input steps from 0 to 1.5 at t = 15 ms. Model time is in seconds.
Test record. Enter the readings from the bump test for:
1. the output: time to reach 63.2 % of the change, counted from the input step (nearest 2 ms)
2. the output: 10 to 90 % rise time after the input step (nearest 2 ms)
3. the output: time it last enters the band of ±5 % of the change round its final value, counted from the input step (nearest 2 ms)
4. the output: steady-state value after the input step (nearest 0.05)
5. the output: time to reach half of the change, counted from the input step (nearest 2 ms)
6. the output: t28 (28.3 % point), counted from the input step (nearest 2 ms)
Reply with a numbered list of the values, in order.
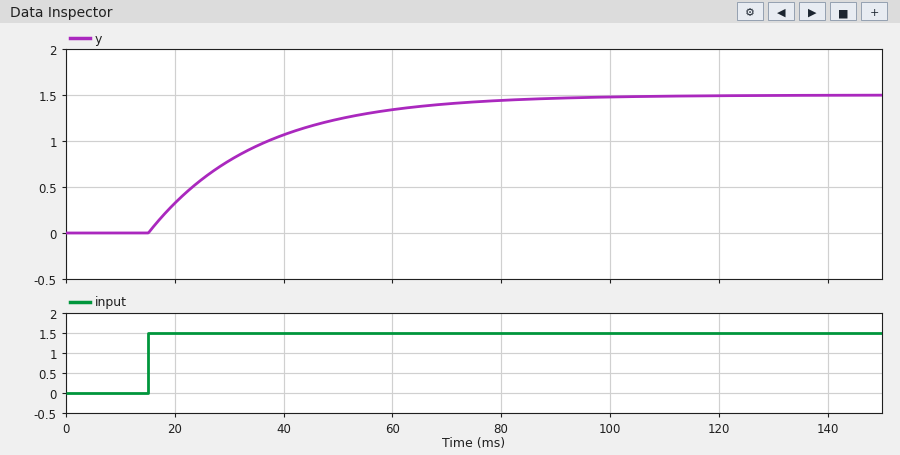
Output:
1. 20 ms
2. 44 ms
3. 60 ms
4. 1.50
5. 14 ms
6. 6 ms
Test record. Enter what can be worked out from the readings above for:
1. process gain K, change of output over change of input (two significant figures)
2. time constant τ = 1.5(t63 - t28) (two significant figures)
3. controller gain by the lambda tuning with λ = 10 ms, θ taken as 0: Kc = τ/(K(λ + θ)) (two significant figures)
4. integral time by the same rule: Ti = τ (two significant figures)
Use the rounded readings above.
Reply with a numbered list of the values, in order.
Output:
1. 1.0
2. 21 ms
3. 2.1
4. 21 ms
